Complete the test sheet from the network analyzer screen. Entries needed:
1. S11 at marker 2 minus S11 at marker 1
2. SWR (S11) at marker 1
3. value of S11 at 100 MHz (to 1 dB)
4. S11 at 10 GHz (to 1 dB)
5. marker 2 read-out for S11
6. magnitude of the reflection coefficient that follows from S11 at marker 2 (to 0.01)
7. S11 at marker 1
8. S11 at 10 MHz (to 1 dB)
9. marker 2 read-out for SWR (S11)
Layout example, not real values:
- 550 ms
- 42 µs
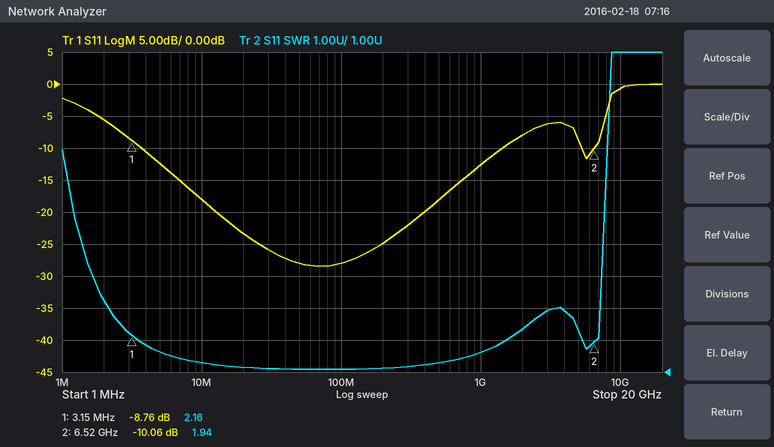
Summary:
- -1.30 dB
- 2.16
- -28 dB
- -1 dB
- -10.06 dB
- 0.31
- -8.76 dB
- -18 dB
- 1.94
